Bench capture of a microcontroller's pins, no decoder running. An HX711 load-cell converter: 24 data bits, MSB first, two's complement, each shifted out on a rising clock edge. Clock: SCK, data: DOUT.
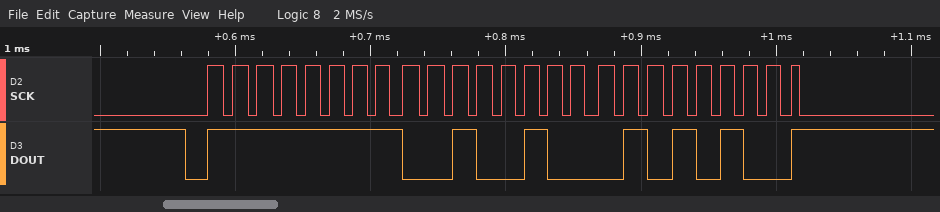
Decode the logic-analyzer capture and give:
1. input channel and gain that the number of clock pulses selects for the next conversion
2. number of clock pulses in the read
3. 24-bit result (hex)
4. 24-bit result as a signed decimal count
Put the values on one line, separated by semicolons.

channel A, gain 128; 25; 0xFF2454; -56236
